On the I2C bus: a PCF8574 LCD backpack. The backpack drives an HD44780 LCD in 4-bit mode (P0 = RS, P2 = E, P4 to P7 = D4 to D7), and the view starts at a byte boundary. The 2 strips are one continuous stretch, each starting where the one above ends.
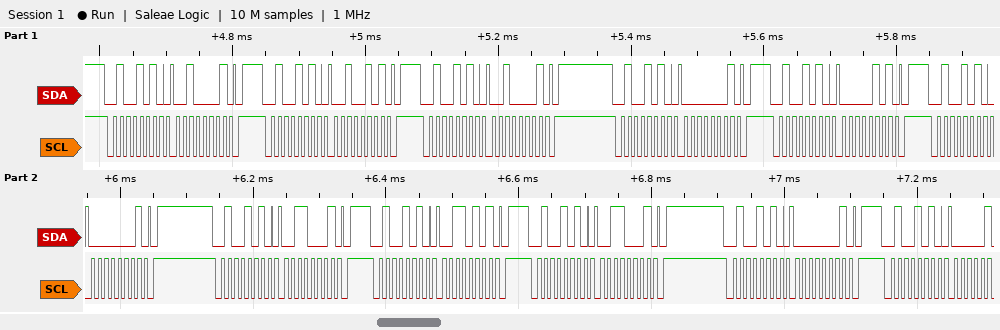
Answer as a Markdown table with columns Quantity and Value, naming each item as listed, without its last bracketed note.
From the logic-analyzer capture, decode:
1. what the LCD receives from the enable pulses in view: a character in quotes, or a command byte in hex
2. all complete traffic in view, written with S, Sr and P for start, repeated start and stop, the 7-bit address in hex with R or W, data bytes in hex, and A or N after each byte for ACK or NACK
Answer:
| Quantity | Value |
|---|---|
| what the LCD receives from the enable pulses in view: a character in quotes, or a command byte in hex | ' ' |
| all complete traffic in view, written with S, Sr and P for start, repeated start and stop, the 7-bit address in hex with R or W, data bytes in hex, and A or N after each byte for ACK or NACK | S 25W A 21 A P S 25W A 25 A P S 25W A 21 A P S 25W A 01 A P S 25W A 05 A P S 25W A 01 A P S 25W A 31 A P S 25W A 35 A P S 25W A 31 A P S 25W A 01 A P S 25W A |
